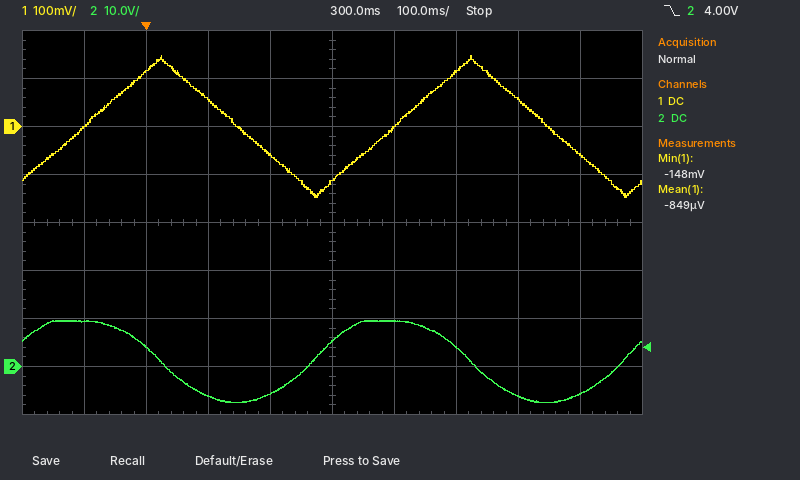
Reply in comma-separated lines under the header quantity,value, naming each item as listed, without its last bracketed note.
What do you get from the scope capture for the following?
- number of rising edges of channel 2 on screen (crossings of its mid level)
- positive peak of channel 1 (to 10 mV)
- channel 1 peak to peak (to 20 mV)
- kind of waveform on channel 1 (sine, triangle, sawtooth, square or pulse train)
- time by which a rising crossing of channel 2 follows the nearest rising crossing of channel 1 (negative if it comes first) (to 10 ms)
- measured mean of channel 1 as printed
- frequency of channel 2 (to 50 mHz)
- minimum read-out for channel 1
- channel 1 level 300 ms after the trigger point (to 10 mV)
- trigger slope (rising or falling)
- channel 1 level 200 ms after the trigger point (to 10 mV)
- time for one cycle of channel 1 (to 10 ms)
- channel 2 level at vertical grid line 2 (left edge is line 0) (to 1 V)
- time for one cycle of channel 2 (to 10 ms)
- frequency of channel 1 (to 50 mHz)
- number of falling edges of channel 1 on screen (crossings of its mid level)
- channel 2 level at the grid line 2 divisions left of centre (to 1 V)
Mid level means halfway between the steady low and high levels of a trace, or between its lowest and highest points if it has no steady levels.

quantity,value
number of rising edges of channel 2 on screen,2
positive peak of channel 1,150 mV
channel 1 peak to peak,300 mV
kind of waveform on channel 1,triangle
time by which a rising crossing of channel 2 follows the nearest rising crossing of channel 1 (negative if it comes first),-130 ms
measured mean of channel 1 as printed,-849 µV
frequency of channel 2,2.00 Hz
minimum read-out for channel 1,-148 mV
channel 1 level 300 ms after the trigger point,-110 mV
trigger slope,falling
channel 1 level 200 ms after the trigger point,-60 mV
time for one cycle of channel 1,500 ms
channel 2 level at vertical grid line 2 (left edge is line 0),4 V
time for one cycle of channel 2,500 ms
frequency of channel 1,2.00 Hz
number of falling edges of channel 1 on screen,2
channel 2 level at the grid line 2 divisions left of centre,-6 V
